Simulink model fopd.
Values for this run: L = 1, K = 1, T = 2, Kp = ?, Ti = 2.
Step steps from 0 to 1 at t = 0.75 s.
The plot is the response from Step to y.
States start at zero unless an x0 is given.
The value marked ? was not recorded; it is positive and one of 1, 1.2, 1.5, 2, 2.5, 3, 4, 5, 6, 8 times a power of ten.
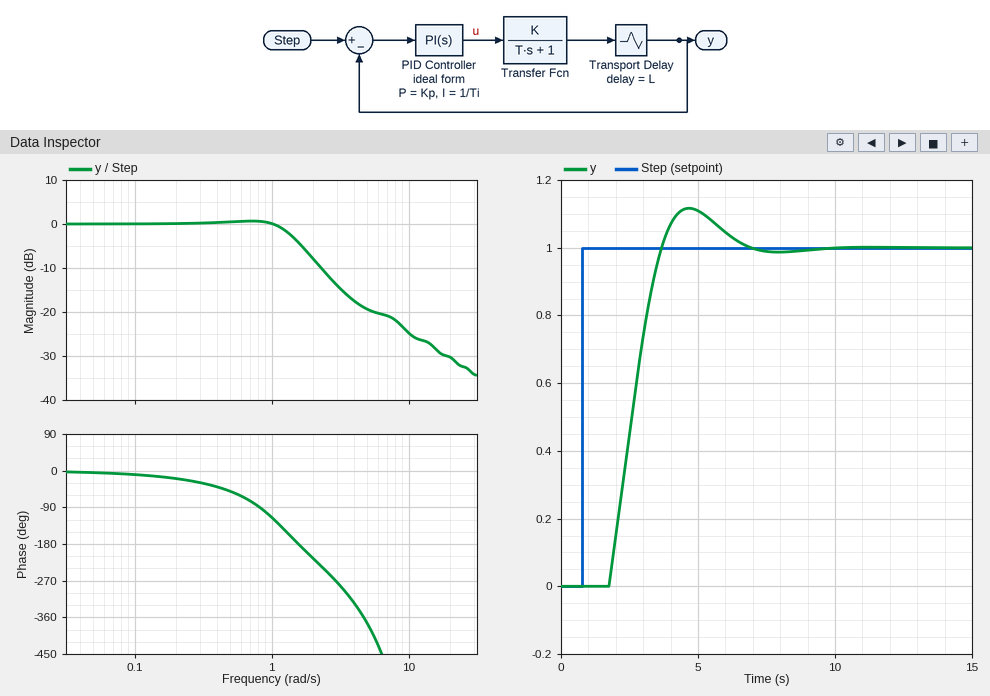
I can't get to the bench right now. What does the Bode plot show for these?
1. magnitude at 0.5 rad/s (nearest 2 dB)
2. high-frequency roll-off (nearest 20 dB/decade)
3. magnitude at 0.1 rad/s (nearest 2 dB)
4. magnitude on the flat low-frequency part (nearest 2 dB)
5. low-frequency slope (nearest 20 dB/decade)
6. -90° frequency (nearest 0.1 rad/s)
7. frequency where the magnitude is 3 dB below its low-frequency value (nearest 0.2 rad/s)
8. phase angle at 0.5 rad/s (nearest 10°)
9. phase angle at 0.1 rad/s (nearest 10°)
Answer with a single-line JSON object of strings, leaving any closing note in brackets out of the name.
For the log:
{"magnitude at 0.5 rad/s": "0 dB", "high-frequency roll-off": "-20 dB/decade", "magnitude at 0.1 rad/s": "0 dB", "magnitude on the flat low-frequency part": "0 dB", "low-frequency slope": "0 dB/decade", "-90° frequency": "0.8 rad/s", "frequency where the magnitude is 3 dB below its low-frequency value": "1.4 rad/s", "phase angle at 0.5 rad/s": "-50°", "phase angle at 0.1 rad/s": "-10°"}
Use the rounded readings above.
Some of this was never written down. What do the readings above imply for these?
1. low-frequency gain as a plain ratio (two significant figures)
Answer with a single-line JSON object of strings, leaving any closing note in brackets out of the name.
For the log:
{"low-frequency gain as a plain ratio": "1.0"}
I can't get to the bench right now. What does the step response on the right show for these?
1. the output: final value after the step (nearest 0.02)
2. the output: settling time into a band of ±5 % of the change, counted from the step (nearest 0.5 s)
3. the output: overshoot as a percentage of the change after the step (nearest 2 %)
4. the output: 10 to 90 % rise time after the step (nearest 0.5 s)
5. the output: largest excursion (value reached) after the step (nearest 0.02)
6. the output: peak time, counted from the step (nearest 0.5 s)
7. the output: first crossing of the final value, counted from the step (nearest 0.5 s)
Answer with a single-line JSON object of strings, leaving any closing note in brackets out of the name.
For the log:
{"the output: final value after the step": "1.00", "the output: settling time into a band of ±5 % of the change, counted from the step": "5.0 s", "the output: overshoot as a percentage of the change after the step": "12 %", "the output: 10 to 90 % rise time after the step": "1.5 s", "the output: largest excursion (value reached) after the step": "1.12", "the output: peak time, counted from the step": "4.0 s", "the output: first crossing of the final value, counted from the step": "3.0 s"}
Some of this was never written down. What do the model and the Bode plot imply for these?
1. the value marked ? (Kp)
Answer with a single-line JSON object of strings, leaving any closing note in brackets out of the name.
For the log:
{"the value marked ?": "1.2"}
